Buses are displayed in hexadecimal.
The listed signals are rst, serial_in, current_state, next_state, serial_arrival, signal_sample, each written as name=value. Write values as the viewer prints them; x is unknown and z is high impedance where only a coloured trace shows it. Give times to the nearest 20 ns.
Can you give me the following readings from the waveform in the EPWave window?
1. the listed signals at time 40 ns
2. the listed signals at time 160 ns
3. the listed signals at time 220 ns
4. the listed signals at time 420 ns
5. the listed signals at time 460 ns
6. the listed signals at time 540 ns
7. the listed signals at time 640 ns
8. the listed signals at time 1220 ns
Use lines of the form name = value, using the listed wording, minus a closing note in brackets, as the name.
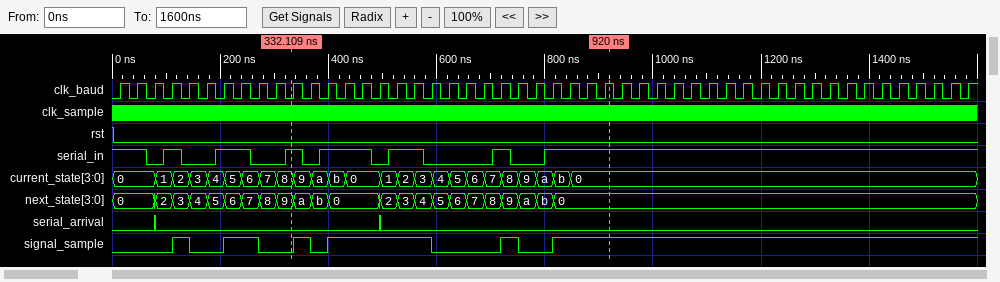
the listed signals at time 40 ns = rst=0, serial_in=1, current_state=0, next_state=0, serial_arrival=0, signal_sample=0
the listed signals at time 160 ns = rst=0, serial_in=0, current_state=3, next_state=4, serial_arrival=0, signal_sample=0
the listed signals at time 220 ns = rst=0, serial_in=1, current_state=5, next_state=6, serial_arrival=0, signal_sample=1
the listed signals at time 420 ns = rst=0, serial_in=1, current_state=b, next_state=0, serial_arrival=0, signal_sample=1
the listed signals at time 460 ns = rst=0, serial_in=1, current_state=0, next_state=0, serial_arrival=0, signal_sample=1
the listed signals at time 540 ns = rst=0, serial_in=1, current_state=2, next_state=3, serial_arrival=0, signal_sample=1
the listed signals at time 640 ns = rst=0, serial_in=0, current_state=5, next_state=6, serial_arrival=0, signal_sample=0
the listed signals at time 1220 ns = rst=0, serial_in=1, current_state=0, next_state=0, serial_arrival=0, signal_sample=1
